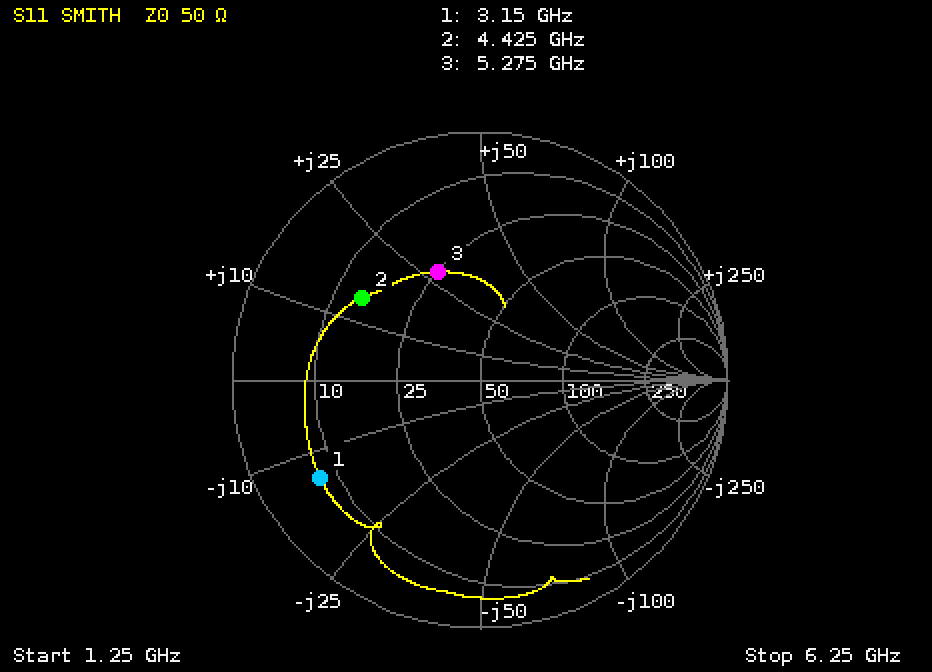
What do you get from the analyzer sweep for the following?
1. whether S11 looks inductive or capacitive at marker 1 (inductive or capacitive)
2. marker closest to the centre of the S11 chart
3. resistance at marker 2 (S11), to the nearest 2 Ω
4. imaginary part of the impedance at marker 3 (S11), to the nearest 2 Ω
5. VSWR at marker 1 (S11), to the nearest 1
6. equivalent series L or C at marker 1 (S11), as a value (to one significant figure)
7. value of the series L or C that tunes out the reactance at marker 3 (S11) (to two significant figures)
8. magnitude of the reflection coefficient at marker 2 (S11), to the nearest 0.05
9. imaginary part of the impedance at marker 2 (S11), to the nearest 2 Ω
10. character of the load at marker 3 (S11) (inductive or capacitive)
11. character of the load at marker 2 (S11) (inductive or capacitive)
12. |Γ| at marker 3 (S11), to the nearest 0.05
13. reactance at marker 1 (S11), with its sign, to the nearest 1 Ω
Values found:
capacitive
marker 3
14 Ω
+28 Ω
7
4 pF
1.1 pF
0.60
+14 Ω
inductive
inductive
0.45
-14 Ω
